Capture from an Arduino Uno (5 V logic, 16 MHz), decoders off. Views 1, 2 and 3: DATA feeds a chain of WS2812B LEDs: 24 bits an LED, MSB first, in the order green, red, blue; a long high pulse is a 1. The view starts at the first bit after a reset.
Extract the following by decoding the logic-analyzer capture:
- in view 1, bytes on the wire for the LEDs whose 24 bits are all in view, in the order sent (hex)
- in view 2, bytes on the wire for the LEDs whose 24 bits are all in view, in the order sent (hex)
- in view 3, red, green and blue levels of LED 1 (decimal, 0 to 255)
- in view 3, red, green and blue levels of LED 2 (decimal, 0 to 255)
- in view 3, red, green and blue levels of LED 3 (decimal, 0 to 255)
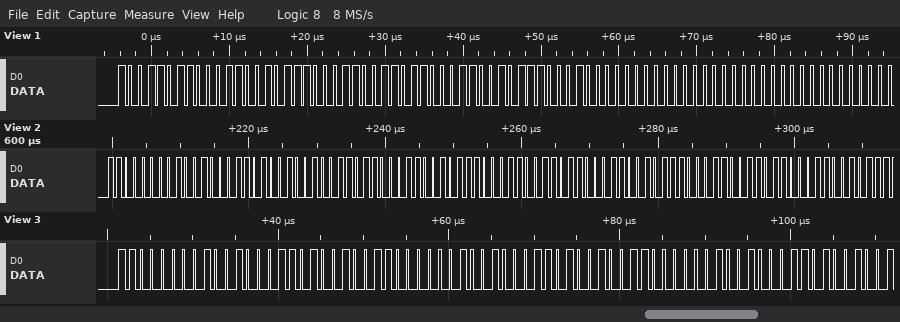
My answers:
9B 19 71 9B 19 71 00 00 00
C0 91 A4 9B 19 71 9B 19 71
145, 192, 164
145, 192, 164
145, 192, 164
